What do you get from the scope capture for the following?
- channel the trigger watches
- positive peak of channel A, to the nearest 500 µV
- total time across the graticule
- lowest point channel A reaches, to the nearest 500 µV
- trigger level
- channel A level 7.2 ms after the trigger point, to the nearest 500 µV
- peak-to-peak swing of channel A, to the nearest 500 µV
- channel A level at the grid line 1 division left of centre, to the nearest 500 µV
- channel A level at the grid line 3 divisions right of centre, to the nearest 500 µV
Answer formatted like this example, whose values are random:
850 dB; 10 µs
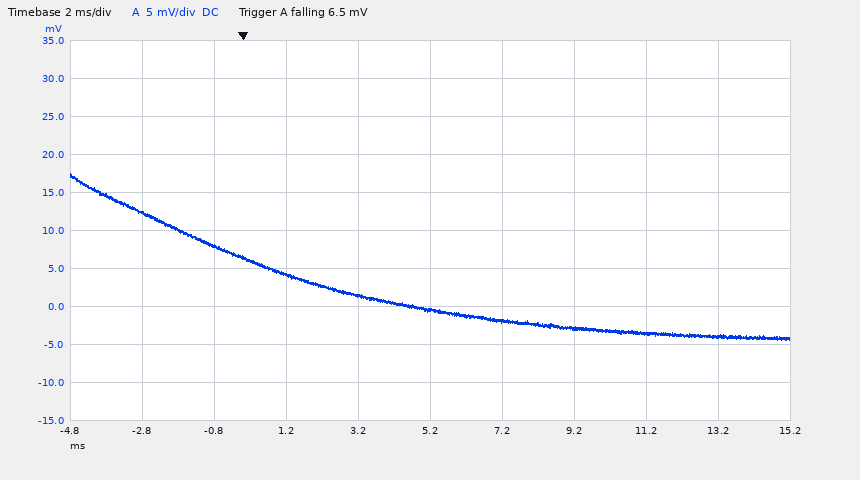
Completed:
channel A; 17.5 mV; 20 ms; -4.5 mV; 6.5 mV; -2.0 mV; 22.0 mV; 1.5 mV; -3.5 mV
